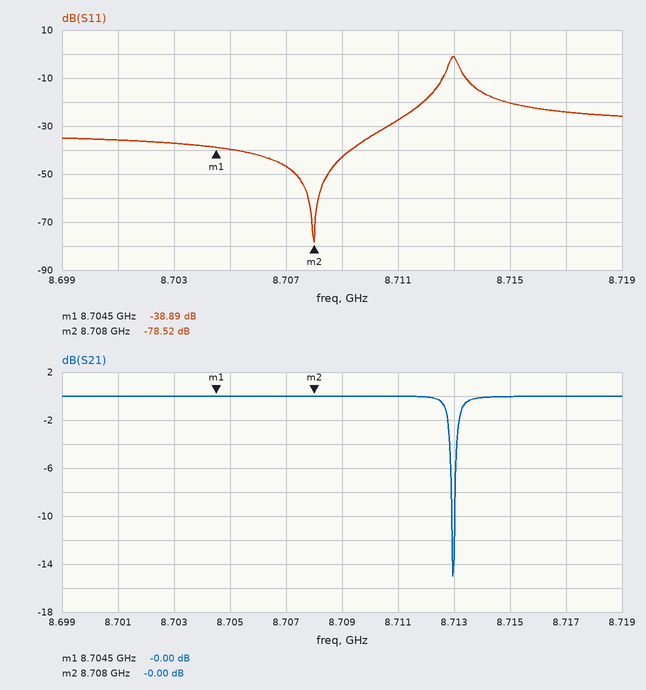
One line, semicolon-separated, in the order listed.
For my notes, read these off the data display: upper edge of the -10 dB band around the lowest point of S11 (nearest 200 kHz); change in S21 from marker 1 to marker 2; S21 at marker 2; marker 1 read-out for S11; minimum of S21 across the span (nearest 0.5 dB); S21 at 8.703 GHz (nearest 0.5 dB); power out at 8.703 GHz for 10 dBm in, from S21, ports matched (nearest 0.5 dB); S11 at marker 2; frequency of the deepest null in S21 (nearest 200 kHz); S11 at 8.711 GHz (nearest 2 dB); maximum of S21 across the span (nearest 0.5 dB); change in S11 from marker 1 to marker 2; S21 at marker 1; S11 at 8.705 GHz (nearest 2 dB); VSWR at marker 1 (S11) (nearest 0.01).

8.7126 GHz; 0.00 dB; -0.00 dB; -38.89 dB; -15.0 dB; 0.0 dB; 10.0 dBm; -78.52 dB; 8.7130 GHz; -28 dB; 0.0 dB; -39.63 dB; -0.00 dB; -40 dB; 1.02
